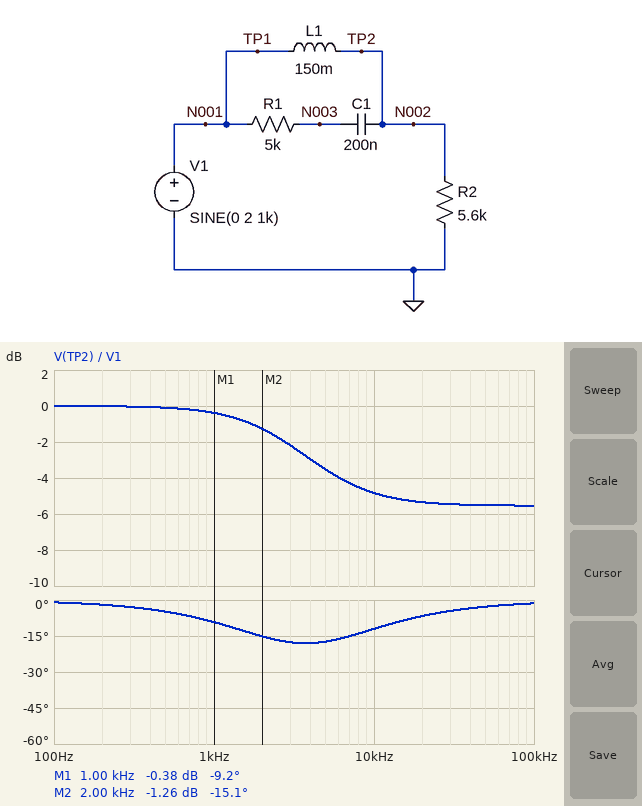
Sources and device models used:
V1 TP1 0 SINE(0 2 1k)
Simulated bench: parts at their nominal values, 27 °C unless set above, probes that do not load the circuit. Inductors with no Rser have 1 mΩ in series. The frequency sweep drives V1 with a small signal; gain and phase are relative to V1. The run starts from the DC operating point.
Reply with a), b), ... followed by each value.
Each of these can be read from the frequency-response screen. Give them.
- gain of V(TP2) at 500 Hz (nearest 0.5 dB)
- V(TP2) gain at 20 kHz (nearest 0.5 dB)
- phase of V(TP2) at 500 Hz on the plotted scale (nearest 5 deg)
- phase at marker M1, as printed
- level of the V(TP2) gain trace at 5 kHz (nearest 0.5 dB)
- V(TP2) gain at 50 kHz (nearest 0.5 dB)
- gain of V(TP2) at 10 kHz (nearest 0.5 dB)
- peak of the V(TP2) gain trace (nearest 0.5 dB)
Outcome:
a) 0 dB
b) -5.5 dB
c) -5 deg
d) -9.2 deg
e) -3.5 dB
f) -5.5 dB
g) -5.0 dB
h) 0 dB
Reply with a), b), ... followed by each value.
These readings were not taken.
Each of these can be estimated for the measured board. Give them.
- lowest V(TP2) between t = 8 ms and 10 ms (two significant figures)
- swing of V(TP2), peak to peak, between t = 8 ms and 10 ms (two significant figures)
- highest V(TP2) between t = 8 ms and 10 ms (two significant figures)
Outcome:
a) -1.9 V
b) 3.8 V
c) 1.9 V
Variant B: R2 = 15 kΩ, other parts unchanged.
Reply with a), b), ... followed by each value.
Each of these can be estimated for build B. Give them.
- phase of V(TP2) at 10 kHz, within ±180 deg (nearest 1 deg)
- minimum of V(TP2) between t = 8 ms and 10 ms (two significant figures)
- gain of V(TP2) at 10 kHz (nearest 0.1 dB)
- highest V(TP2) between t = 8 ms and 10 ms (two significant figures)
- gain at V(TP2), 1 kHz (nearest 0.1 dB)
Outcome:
a) -6 deg
b) -2.0 V
c) -2.1 dB
d) 2.0 V
e) -0.1 dB
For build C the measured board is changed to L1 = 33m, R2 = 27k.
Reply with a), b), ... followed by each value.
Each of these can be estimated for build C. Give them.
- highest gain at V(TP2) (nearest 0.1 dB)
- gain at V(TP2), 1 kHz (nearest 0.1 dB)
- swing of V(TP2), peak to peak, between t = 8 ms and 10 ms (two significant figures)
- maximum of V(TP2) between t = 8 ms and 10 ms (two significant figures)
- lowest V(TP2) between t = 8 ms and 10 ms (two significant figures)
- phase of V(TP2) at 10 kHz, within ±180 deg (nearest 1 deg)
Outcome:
a) 0 dB
b) 0 dB
c) 4.0 V
d) 2.0 V
e) -2.0 V
f) -4 deg
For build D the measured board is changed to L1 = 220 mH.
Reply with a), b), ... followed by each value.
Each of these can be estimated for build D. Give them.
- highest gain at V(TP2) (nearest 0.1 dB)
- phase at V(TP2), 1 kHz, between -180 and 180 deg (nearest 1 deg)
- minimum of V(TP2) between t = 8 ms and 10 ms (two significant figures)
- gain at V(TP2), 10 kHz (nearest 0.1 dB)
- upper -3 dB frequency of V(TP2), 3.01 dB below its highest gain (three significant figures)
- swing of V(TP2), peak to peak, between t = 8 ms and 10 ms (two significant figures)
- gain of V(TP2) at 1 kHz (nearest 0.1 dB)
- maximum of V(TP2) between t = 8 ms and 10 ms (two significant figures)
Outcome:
a) 0 dB
b) -13 deg
c) -1.8 V
d) -5.2 dB
e) 2.75 kHz
f) 3.7 V
g) -0.8 dB
h) 1.8 V
